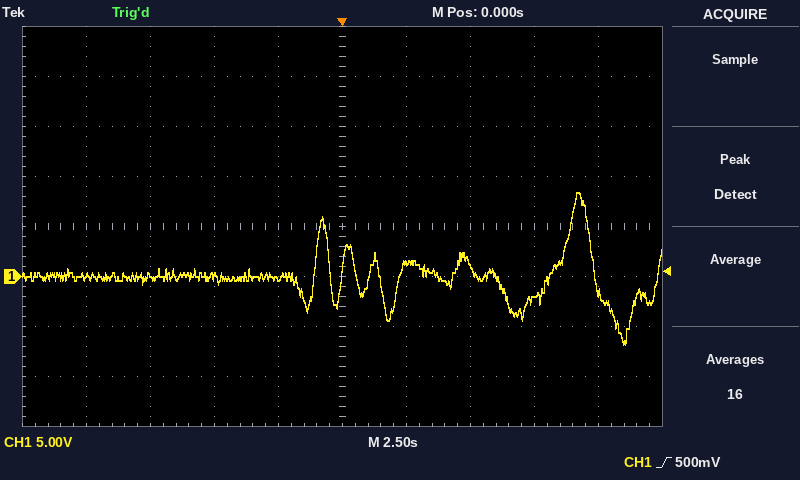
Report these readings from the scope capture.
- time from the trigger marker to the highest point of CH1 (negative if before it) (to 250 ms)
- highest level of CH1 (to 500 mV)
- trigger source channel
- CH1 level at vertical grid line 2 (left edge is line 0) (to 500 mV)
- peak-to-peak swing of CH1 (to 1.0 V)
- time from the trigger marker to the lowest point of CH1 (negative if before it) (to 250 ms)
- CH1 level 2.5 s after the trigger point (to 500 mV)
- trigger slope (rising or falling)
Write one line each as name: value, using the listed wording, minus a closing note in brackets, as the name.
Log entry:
time from the trigger marker to the highest point of CH1 (negative if before it): +9.25 s
highest level of CH1: 8.5 V
trigger source channel: CH1
CH1 level at vertical grid line 2 (left edge is line 0): 0.0 V
peak-to-peak swing of CH1: 15.0 V
time from the trigger marker to the lowest point of CH1 (negative if before it): +11.00 s
CH1 level 2.5 s after the trigger point: 1.5 V
trigger slope: rising
